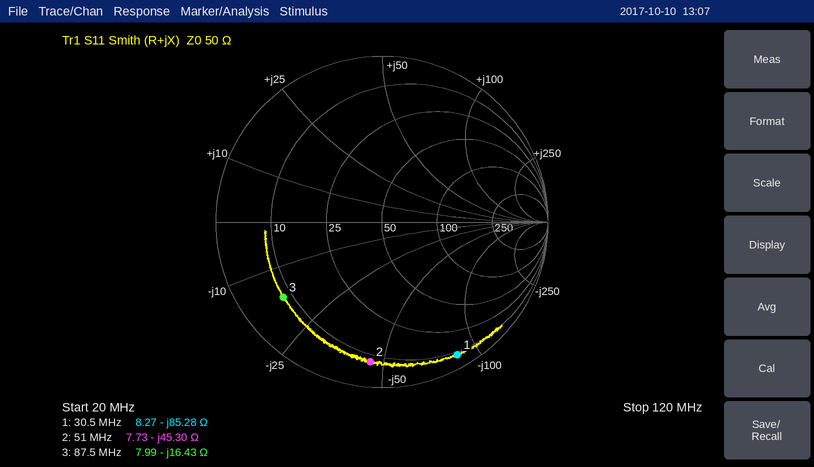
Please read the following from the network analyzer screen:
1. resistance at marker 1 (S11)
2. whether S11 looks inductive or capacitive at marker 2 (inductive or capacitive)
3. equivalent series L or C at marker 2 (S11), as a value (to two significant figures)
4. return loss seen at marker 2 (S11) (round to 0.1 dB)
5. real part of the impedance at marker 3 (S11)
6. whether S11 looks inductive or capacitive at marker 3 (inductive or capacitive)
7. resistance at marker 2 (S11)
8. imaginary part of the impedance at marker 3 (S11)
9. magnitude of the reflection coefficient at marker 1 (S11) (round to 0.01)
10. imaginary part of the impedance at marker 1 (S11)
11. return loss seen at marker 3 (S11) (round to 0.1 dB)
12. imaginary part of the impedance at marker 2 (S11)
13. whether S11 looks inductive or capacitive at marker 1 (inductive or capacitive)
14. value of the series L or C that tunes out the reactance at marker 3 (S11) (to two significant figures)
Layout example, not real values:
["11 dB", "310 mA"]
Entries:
["8.27 Ω", "capacitive", "69 pF", "1.5 dB", "7.99 Ω", "capacitive", "7.73 Ω", "-16.43 Ω", "0.92", "-85.28 Ω", "2.5 dB", "-45.30 Ω", "capacitive", "30 nH"]
